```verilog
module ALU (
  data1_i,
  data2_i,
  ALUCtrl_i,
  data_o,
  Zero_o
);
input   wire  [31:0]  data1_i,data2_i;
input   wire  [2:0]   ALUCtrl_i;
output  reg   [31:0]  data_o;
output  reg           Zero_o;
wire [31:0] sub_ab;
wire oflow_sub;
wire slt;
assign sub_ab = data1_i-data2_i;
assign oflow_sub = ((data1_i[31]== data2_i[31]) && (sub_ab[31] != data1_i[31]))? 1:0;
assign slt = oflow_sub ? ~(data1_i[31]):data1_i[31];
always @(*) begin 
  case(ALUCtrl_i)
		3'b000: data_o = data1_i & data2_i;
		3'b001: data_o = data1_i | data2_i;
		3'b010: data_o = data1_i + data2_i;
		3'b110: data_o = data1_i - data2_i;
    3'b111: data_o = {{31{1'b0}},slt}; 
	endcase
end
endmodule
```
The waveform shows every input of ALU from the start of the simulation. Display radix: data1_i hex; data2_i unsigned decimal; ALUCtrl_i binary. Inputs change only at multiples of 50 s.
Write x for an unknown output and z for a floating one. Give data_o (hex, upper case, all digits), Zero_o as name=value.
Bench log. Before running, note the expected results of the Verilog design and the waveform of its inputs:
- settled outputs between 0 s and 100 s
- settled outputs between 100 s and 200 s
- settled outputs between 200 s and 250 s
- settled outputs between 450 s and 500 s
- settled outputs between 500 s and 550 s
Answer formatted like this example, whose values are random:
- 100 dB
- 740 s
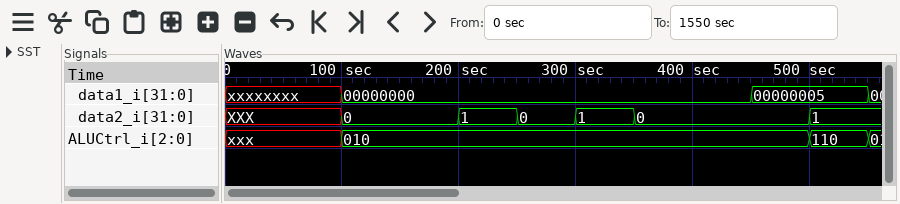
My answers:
- data_o=x, Zero_o=x
- data_o=00000000, Zero_o=x
- data_o=00000001, Zero_o=x
- data_o=00000005, Zero_o=x
- data_o=00000004, Zero_o=x
